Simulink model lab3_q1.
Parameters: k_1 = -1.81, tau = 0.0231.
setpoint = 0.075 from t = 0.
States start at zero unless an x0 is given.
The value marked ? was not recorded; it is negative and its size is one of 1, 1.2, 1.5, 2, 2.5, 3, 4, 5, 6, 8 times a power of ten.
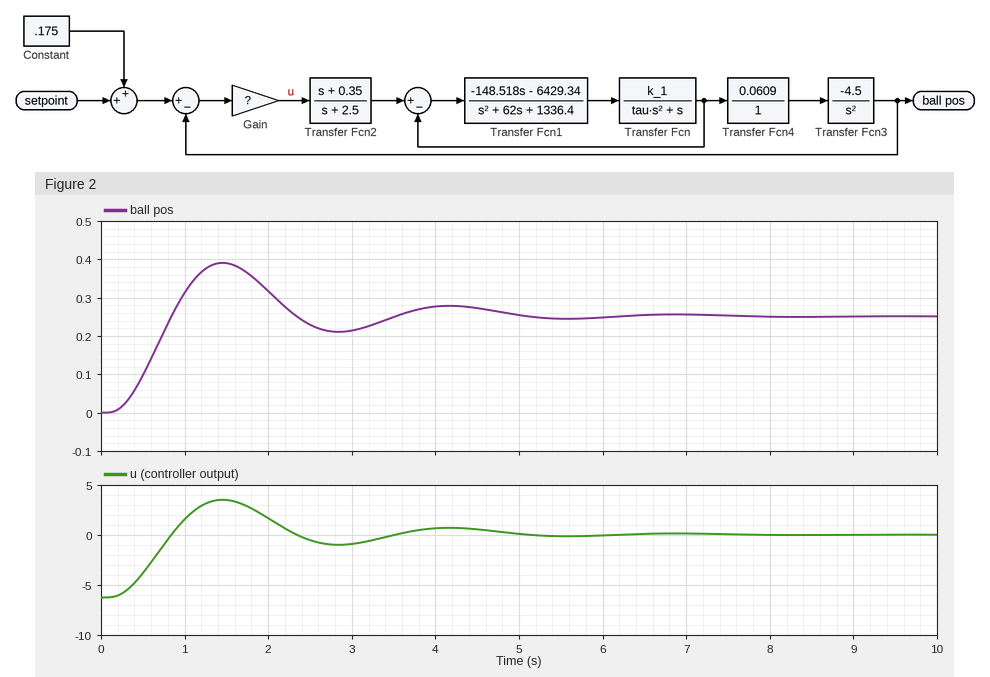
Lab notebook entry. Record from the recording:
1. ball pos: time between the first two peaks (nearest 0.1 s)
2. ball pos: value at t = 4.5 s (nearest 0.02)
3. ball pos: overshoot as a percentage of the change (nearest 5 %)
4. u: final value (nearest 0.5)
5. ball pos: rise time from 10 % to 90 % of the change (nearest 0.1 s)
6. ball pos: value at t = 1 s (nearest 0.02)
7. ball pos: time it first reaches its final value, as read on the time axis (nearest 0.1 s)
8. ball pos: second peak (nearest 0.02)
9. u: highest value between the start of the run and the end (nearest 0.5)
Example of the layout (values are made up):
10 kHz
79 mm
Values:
2.7 s
0.28
55 %
0.0
0.5 s
0.32
0.8 s
0.28
3.5
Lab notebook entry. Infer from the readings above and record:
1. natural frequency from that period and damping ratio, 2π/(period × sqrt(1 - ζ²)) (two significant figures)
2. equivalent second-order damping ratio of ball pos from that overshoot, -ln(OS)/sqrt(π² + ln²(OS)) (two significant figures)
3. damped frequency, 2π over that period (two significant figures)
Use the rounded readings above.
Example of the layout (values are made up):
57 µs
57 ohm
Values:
2.4 rad/s
0.19
2.3 rad/s
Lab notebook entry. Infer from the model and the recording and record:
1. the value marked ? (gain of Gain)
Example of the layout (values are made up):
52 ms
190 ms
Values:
-25
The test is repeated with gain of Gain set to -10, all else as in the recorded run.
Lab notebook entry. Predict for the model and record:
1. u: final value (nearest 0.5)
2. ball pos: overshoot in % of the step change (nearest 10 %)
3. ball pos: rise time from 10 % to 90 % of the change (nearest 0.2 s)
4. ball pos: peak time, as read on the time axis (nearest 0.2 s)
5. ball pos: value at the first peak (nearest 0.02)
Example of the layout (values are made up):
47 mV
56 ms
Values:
0.0
40 %
1.0 s
2.6 s
0.34
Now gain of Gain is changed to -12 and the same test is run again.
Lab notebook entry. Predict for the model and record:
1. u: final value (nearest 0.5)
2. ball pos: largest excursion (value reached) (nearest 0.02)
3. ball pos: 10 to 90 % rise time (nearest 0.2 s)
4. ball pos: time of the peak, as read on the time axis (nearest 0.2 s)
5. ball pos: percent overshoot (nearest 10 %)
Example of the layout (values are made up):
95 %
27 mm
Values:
0.0
0.34
0.8 s
2.4 s
40 %
